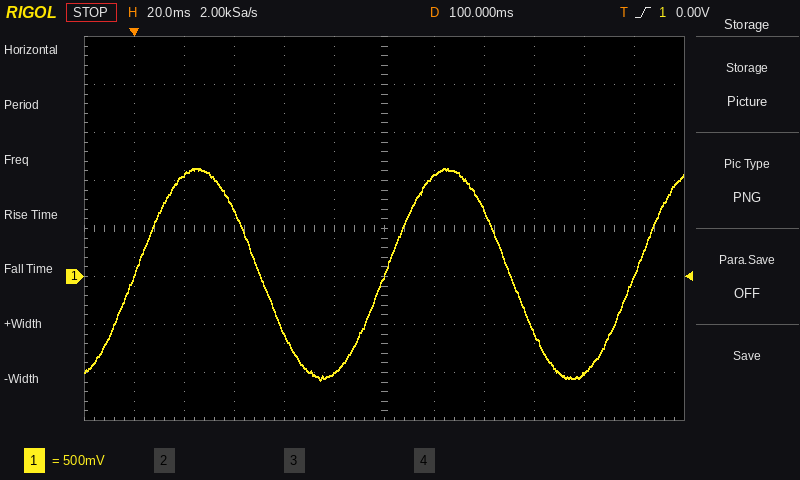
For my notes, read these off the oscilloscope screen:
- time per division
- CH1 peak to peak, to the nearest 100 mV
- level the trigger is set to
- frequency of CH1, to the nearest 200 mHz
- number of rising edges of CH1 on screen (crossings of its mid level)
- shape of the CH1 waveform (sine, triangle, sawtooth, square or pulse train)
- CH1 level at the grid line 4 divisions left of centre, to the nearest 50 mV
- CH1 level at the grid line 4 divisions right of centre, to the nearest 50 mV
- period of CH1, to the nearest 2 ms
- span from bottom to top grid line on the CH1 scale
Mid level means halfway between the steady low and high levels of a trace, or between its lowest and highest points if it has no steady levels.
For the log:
20 ms
2.20 V
0.00 V
10.0 Hz
3
sine
1.05 V
-1.00 V
100 ms
4 V
